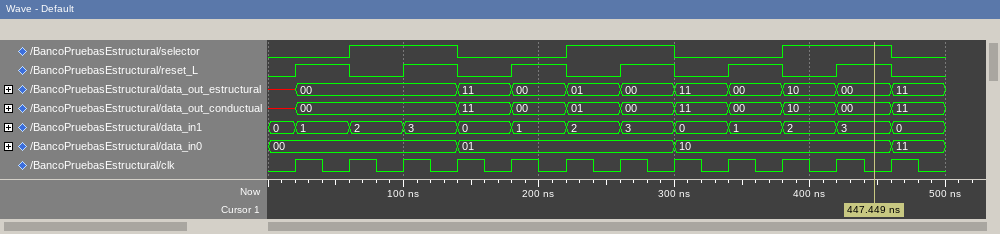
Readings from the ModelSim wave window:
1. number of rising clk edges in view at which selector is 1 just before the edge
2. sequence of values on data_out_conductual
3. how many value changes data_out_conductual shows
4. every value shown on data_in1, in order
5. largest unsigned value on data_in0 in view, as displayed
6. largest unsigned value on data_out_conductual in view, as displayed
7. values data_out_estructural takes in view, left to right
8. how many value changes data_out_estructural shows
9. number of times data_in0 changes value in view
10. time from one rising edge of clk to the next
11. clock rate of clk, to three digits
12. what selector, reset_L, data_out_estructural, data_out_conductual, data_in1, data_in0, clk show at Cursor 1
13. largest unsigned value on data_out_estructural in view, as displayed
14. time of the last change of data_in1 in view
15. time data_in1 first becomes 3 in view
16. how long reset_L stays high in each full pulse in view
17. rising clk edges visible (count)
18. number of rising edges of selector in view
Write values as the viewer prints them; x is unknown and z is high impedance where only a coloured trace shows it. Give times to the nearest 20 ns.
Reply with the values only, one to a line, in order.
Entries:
6
x, 00, 11, 00, 01, 00, 11, 00, 10, 00, 11
10
0, 1, 2, 3, 0, 1, 2, 3, 0, 1, 2, 3, 0
11
11
x, 00, 11, 00, 01, 00, 11, 00, 10, 00, 11
10
3
40 ns
25.0 MHz
selector=1, reset_L=1, data_out_estructural=00, data_out_conductual=00, data_in1=3, data_in0=10, clk=0
11
460 ns
100 ns
40 ns, 40 ns, 40 ns, 40 ns, 40 ns, 40 ns
12
3
